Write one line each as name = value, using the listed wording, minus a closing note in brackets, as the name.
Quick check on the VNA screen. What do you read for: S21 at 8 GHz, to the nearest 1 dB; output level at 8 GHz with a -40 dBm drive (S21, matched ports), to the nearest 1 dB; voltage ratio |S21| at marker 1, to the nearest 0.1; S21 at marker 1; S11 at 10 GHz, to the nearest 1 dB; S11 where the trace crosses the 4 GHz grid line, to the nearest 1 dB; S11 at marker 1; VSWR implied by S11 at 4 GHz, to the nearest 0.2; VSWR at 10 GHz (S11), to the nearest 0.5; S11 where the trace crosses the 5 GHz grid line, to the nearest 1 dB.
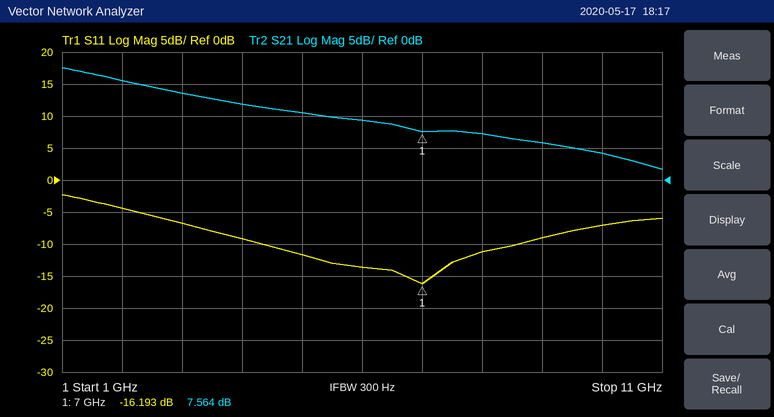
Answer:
S21 at 8 GHz, to the nearest 1 dB = 7 dB
output level at 8 GHz with a -40 dBm drive (S21, matched ports), to the nearest 1 dB = -33 dBm
voltage ratio |S21| at marker 1, to the nearest 0.1 = 2.4
S21 at marker 1 = 7.564 dB
S11 at 10 GHz, to the nearest 1 dB = -7 dB
S11 where the trace crosses the 4 GHz grid line, to the nearest 1 dB = -9 dB
S11 at marker 1 = -16.193 dB
VSWR implied by S11 at 4 GHz, to the nearest 0.2 = 2.0
VSWR at 10 GHz (S11), to the nearest 0.5 = 2.5
S11 where the trace crosses the 5 GHz grid line, to the nearest 1 dB = -12 dB
